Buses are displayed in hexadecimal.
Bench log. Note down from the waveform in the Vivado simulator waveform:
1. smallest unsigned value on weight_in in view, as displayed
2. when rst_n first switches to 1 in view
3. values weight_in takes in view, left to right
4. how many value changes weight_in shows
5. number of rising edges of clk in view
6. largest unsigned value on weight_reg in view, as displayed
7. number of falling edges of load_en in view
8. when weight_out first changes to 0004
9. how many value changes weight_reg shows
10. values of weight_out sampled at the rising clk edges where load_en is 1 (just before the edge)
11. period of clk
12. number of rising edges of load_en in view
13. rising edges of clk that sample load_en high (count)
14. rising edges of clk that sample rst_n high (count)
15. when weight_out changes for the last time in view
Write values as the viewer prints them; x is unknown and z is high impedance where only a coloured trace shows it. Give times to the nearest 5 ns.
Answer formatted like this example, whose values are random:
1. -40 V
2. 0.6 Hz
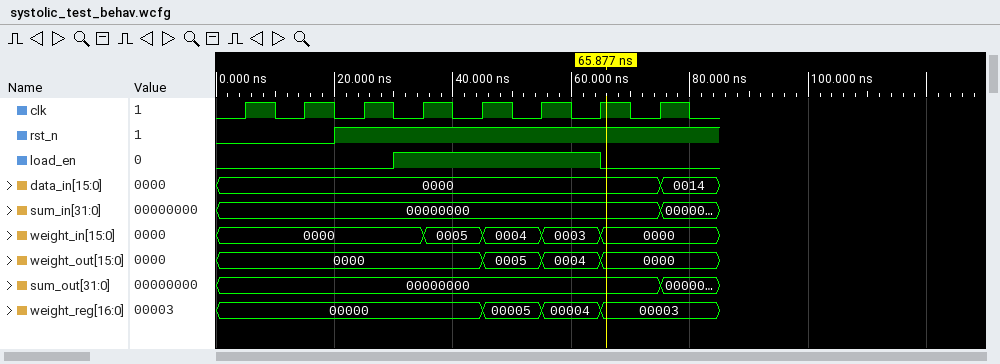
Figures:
1. 0000
2. 20 ns
3. 0000, 0005, 0004, 0003, 0000
4. 4
5. 8
6. 00005
7. 1
8. 55 ns
9. 3
10. 0000, 0000, 0005, 0004
11. 10 ns
12. 1
13. 4
14. 6
15. 65 ns
